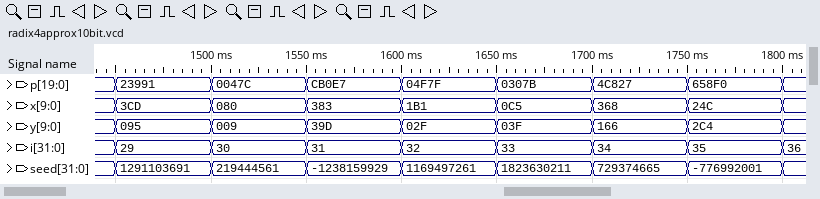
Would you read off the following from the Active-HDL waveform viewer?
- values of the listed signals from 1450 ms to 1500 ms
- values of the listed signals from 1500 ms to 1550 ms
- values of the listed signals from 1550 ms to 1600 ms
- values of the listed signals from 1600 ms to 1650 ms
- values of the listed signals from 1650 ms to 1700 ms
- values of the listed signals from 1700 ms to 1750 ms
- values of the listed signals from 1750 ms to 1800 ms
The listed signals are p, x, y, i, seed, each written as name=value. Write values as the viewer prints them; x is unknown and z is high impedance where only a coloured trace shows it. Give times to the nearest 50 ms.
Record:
p=23991, x=3CD, y=095, i=29, seed=1291103691
p=0047C, x=080, y=009, i=30, seed=219444561
p=CB0E7, x=383, y=39D, i=31, seed=-1238159929
p=04F7F, x=1B1, y=02F, i=32, seed=1169497261
p=0307B, x=0C5, y=03F, i=33, seed=1823630211
p=4C827, x=368, y=166, i=34, seed=729374665
p=658F0, x=24C, y=2C4, i=35, seed=-776992001
